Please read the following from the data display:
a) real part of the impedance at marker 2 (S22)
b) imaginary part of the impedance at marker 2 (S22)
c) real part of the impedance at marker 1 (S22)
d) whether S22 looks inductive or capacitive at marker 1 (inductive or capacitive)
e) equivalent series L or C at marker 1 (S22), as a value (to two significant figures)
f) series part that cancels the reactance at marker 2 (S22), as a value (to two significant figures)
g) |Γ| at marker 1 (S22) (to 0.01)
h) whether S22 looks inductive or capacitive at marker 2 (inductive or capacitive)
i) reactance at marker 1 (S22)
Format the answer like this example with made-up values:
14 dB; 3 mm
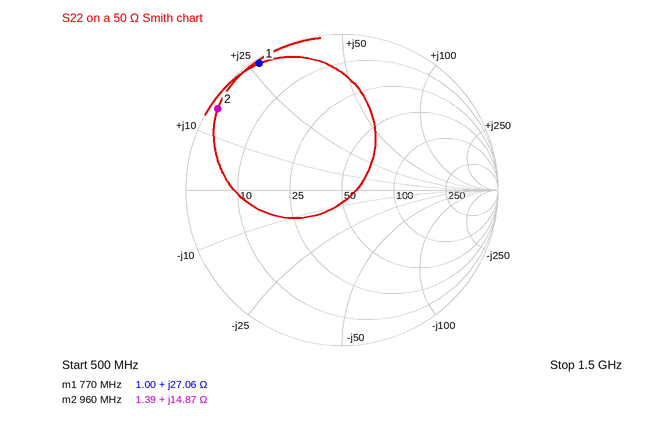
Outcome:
1.39 Ω; +14.87 Ω; 1.00 Ω; inductive; 5.6 nH; 11 pF; 0.97; inductive; +27.06 Ω
